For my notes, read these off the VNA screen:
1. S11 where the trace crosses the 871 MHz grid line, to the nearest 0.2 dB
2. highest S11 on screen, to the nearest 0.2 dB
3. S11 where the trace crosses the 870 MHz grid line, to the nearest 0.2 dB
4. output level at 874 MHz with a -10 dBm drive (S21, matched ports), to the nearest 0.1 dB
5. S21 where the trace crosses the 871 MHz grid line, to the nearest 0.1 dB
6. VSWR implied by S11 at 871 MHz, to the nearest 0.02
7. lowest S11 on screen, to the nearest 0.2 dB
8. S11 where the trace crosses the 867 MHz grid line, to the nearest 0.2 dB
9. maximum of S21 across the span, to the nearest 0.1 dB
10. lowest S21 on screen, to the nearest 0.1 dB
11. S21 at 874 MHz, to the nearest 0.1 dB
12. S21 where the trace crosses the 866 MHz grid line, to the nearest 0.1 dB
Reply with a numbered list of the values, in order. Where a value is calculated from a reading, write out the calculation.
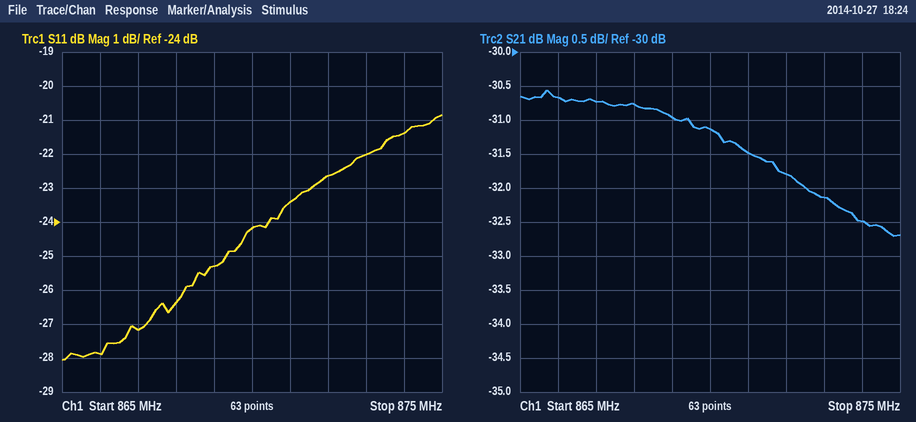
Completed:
1. -23.4 dB
2. -20.8 dB
3. -24.2 dB
4. -10 dBm + (-32.5 dB) = -42.5 dBm
5. -31.5 dB
6. |Γ| = 10^(-23.4/20) = 0.0676; VSWR = (1 + 0.0676)/(1 − 0.0676) ≈ 1.15, so 1.14 to the nearest 0.02
7. -28.0 dB
8. -27.2 dB
9. -30.6 dB
10. -32.7 dB
11. -32.5 dB
12. -30.7 dB
